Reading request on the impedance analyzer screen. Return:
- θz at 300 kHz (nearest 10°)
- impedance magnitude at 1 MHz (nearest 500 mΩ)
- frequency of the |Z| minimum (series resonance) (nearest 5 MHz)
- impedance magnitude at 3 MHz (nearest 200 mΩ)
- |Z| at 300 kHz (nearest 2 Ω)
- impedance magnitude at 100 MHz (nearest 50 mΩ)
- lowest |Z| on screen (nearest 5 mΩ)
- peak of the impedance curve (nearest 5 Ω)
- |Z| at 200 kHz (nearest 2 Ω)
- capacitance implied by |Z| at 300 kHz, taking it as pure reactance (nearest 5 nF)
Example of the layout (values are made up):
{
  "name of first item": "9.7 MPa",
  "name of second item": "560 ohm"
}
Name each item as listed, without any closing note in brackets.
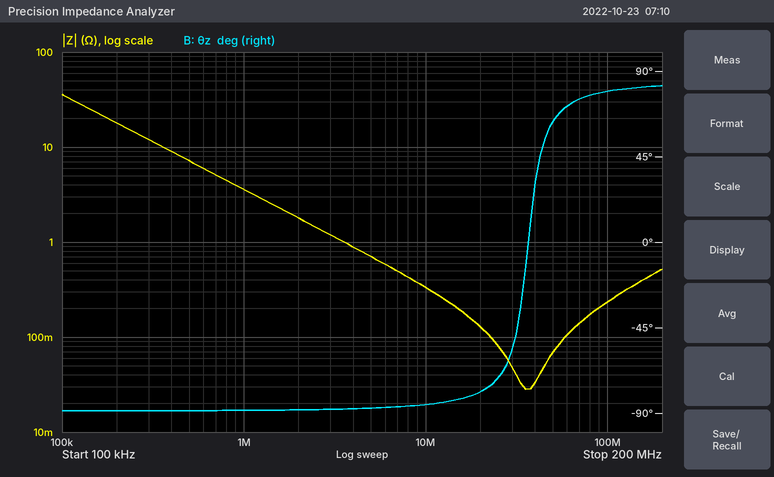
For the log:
{
  "θz at 300 kHz": "-90°",
  "impedance magnitude at 1 MHz": "3.5 Ω",
  "frequency of the |Z| minimum (series resonance)": "35 MHz",
  "impedance magnitude at 3 MHz": "1.2 Ω",
  "|Z| at 300 kHz": "12 Ω",
  "impedance magnitude at 100 MHz": "250 mΩ",
  "lowest |Z| on screen": "30 mΩ",
  "peak of the impedance curve": "35 Ω",
  "|Z| at 200 kHz": "18 Ω",
  "capacitance implied by |Z| at 300 kHz, taking it as pure reactance": "45 nF"
}
